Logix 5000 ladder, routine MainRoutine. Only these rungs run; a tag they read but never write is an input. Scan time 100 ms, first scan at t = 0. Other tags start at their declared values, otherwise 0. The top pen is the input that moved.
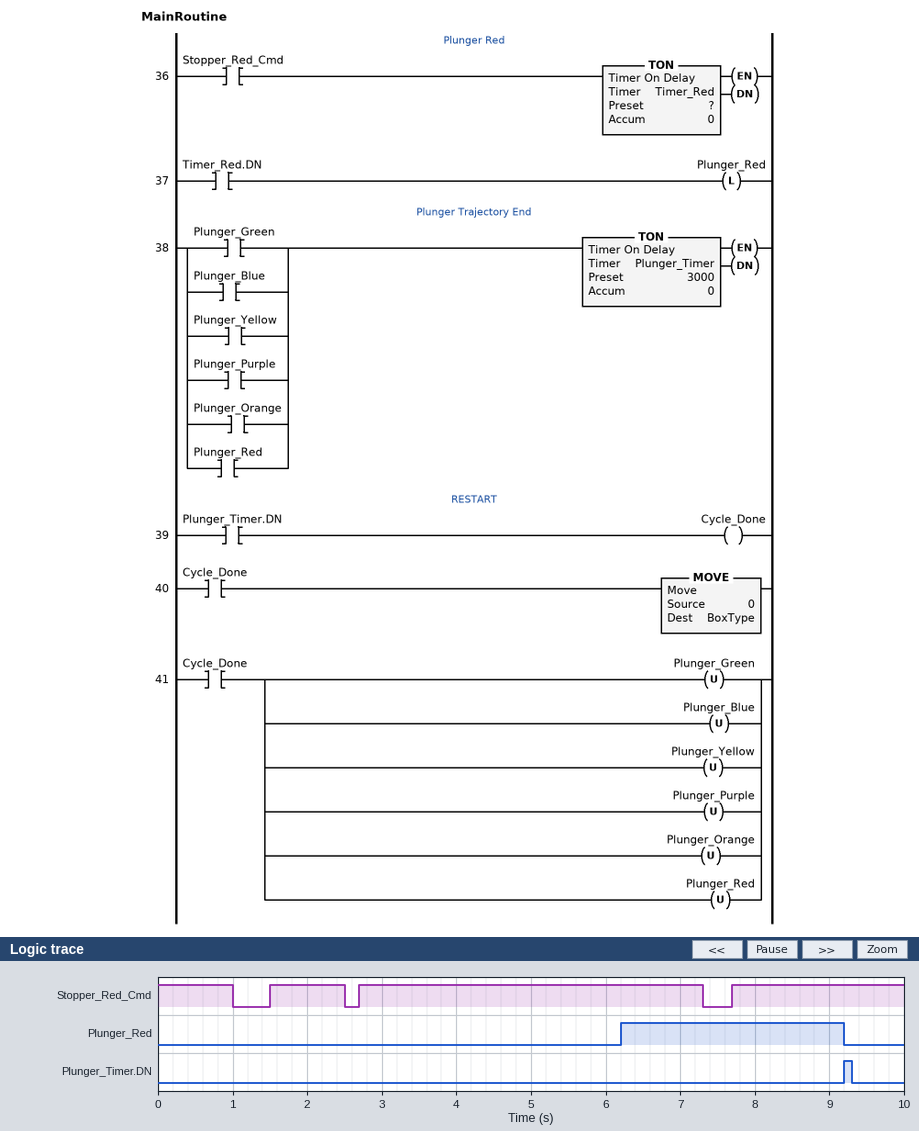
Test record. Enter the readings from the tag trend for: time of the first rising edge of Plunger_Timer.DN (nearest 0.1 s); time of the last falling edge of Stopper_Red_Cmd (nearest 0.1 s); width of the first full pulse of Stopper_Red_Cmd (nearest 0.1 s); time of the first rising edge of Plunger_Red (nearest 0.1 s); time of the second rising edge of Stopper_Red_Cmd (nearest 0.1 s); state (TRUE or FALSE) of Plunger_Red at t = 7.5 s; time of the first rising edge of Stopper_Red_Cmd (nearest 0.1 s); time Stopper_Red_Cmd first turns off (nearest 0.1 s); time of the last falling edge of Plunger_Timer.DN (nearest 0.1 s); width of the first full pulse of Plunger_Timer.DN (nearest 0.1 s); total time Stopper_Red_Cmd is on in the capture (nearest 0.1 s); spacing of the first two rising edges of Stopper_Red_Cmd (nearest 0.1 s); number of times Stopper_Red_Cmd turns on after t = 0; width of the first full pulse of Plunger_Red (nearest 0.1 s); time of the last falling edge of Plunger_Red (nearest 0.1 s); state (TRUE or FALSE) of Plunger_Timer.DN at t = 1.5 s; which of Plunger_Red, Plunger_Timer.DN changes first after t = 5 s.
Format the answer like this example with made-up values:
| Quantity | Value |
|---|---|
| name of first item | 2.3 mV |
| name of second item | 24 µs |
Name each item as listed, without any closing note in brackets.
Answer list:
| Quantity | Value |
|---|---|
| time of the first rising edge of Plunger_Timer.DN | 9.2 s |
| time of the last falling edge of Stopper_Red_Cmd | 7.3 s |
| width of the first full pulse of Stopper_Red_Cmd | 1.0 s |
| time of the first rising edge of Plunger_Red | 6.2 s |
| time of the second rising edge of Stopper_Red_Cmd | 2.7 s |
| state (TRUE or FALSE) of Plunger_Red at t = 7.5 s | TRUE |
| time of the first rising edge of Stopper_Red_Cmd | 1.5 s |
| time Stopper_Red_Cmd first turns off | 1.0 s |
| time of the last falling edge of Plunger_Timer.DN | 9.3 s |
| width of the first full pulse of Plunger_Timer.DN | 0.1 s |
| total time Stopper_Red_Cmd is on in the capture | 8.9 s |
| spacing of the first two rising edges of Stopper_Red_Cmd | 1.2 s |
| number of times Stopper_Red_Cmd turns on after t = 0 | 3 |
| width of the first full pulse of Plunger_Red | 3.0 s |
| time of the last falling edge of Plunger_Red | 9.2 s |
| state (TRUE or FALSE) of Plunger_Timer.DN at t = 1.5 s | FALSE |
| which of Plunger_Red, Plunger_Timer.DN changes first after t = 5 s | Plunger_Red |
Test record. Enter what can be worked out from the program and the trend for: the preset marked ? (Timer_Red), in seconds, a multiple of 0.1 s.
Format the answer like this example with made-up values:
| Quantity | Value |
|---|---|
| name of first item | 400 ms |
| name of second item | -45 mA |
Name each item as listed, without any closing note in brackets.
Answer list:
| Quantity | Value |
|---|---|
| the preset marked ? (Timer_Red), in seconds, a multiple of 0.1 s | 3.5 s |
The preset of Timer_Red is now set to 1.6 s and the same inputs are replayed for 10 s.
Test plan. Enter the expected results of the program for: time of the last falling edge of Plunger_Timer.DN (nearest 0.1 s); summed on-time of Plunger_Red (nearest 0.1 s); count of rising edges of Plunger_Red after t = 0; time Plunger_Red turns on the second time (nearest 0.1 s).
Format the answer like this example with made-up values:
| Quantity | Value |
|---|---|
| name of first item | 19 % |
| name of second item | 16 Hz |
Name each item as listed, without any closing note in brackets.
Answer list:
| Quantity | Value |
|---|---|
| time of the last falling edge of Plunger_Timer.DN | 7.4 s |
| summed on-time of Plunger_Red | 3.7 s |
| count of rising edges of Plunger_Red after t = 0 | 2 |
| time Plunger_Red turns on the second time | 9.3 s |
